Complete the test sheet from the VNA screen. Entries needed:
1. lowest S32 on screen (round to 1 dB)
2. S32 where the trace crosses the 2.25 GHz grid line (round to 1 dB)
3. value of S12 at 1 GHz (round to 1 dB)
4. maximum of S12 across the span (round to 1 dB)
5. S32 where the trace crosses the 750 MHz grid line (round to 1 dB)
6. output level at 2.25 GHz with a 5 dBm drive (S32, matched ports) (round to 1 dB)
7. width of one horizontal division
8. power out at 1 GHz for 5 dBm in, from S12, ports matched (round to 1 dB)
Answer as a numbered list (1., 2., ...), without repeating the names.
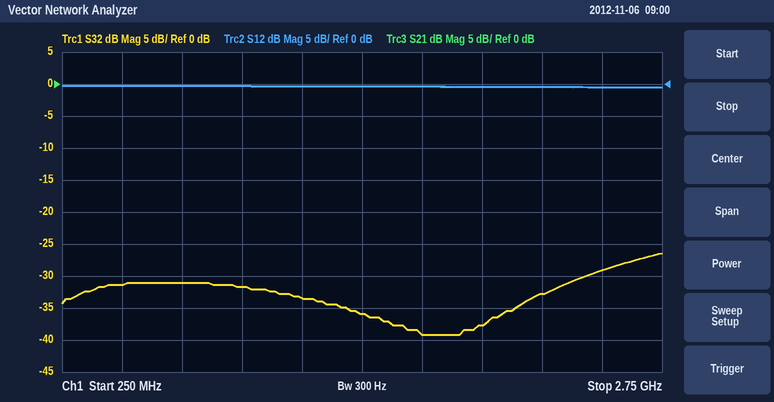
1. -39 dB
2. -33 dB
3. 0 dB
4. 0 dB
5. -31 dB
6. -28 dBm
7. 250 MHz
8. 5 dBm
